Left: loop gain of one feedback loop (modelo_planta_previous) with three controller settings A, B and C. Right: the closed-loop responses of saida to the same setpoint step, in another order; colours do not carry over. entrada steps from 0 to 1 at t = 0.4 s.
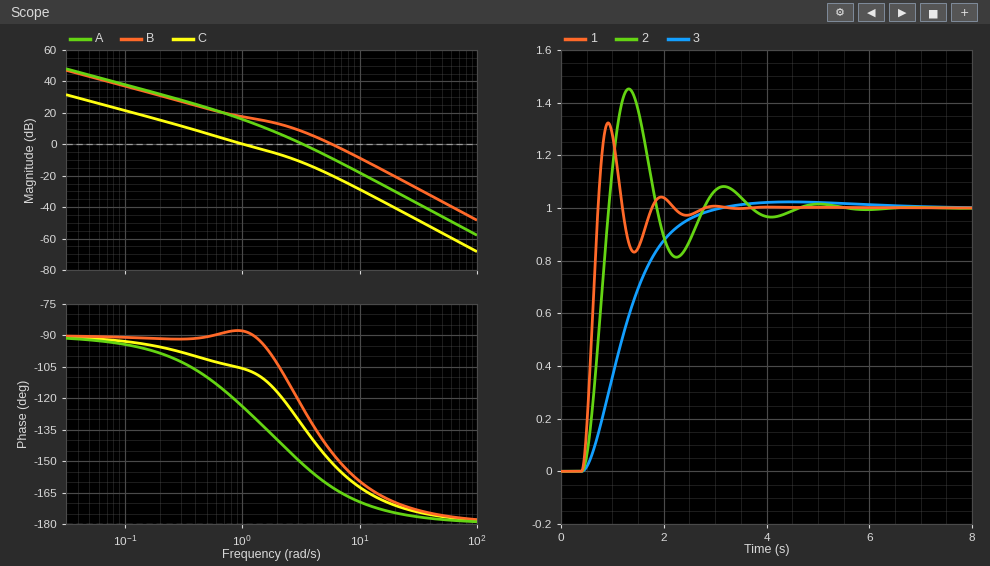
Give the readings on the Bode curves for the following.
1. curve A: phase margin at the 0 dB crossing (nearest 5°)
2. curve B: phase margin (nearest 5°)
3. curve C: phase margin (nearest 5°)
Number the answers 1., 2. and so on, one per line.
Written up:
1. 30°
2. 35°
3. 75°
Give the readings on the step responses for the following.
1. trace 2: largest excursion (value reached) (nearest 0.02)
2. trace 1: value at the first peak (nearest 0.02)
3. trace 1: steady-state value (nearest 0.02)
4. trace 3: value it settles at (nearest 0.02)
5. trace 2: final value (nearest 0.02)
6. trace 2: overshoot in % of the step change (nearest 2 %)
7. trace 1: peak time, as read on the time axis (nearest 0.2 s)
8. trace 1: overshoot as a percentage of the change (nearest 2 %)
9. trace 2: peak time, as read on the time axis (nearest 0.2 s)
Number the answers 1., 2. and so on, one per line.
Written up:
1. 1.46
2. 1.32
3. 1.00
4. 1.00
5. 1.00
6. 46 %
7. 1.0 s
8. 32 %
9. 1.4 s
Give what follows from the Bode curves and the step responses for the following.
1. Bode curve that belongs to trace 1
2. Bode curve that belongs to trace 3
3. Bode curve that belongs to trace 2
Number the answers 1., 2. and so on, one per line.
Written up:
1. B
2. C
3. A
